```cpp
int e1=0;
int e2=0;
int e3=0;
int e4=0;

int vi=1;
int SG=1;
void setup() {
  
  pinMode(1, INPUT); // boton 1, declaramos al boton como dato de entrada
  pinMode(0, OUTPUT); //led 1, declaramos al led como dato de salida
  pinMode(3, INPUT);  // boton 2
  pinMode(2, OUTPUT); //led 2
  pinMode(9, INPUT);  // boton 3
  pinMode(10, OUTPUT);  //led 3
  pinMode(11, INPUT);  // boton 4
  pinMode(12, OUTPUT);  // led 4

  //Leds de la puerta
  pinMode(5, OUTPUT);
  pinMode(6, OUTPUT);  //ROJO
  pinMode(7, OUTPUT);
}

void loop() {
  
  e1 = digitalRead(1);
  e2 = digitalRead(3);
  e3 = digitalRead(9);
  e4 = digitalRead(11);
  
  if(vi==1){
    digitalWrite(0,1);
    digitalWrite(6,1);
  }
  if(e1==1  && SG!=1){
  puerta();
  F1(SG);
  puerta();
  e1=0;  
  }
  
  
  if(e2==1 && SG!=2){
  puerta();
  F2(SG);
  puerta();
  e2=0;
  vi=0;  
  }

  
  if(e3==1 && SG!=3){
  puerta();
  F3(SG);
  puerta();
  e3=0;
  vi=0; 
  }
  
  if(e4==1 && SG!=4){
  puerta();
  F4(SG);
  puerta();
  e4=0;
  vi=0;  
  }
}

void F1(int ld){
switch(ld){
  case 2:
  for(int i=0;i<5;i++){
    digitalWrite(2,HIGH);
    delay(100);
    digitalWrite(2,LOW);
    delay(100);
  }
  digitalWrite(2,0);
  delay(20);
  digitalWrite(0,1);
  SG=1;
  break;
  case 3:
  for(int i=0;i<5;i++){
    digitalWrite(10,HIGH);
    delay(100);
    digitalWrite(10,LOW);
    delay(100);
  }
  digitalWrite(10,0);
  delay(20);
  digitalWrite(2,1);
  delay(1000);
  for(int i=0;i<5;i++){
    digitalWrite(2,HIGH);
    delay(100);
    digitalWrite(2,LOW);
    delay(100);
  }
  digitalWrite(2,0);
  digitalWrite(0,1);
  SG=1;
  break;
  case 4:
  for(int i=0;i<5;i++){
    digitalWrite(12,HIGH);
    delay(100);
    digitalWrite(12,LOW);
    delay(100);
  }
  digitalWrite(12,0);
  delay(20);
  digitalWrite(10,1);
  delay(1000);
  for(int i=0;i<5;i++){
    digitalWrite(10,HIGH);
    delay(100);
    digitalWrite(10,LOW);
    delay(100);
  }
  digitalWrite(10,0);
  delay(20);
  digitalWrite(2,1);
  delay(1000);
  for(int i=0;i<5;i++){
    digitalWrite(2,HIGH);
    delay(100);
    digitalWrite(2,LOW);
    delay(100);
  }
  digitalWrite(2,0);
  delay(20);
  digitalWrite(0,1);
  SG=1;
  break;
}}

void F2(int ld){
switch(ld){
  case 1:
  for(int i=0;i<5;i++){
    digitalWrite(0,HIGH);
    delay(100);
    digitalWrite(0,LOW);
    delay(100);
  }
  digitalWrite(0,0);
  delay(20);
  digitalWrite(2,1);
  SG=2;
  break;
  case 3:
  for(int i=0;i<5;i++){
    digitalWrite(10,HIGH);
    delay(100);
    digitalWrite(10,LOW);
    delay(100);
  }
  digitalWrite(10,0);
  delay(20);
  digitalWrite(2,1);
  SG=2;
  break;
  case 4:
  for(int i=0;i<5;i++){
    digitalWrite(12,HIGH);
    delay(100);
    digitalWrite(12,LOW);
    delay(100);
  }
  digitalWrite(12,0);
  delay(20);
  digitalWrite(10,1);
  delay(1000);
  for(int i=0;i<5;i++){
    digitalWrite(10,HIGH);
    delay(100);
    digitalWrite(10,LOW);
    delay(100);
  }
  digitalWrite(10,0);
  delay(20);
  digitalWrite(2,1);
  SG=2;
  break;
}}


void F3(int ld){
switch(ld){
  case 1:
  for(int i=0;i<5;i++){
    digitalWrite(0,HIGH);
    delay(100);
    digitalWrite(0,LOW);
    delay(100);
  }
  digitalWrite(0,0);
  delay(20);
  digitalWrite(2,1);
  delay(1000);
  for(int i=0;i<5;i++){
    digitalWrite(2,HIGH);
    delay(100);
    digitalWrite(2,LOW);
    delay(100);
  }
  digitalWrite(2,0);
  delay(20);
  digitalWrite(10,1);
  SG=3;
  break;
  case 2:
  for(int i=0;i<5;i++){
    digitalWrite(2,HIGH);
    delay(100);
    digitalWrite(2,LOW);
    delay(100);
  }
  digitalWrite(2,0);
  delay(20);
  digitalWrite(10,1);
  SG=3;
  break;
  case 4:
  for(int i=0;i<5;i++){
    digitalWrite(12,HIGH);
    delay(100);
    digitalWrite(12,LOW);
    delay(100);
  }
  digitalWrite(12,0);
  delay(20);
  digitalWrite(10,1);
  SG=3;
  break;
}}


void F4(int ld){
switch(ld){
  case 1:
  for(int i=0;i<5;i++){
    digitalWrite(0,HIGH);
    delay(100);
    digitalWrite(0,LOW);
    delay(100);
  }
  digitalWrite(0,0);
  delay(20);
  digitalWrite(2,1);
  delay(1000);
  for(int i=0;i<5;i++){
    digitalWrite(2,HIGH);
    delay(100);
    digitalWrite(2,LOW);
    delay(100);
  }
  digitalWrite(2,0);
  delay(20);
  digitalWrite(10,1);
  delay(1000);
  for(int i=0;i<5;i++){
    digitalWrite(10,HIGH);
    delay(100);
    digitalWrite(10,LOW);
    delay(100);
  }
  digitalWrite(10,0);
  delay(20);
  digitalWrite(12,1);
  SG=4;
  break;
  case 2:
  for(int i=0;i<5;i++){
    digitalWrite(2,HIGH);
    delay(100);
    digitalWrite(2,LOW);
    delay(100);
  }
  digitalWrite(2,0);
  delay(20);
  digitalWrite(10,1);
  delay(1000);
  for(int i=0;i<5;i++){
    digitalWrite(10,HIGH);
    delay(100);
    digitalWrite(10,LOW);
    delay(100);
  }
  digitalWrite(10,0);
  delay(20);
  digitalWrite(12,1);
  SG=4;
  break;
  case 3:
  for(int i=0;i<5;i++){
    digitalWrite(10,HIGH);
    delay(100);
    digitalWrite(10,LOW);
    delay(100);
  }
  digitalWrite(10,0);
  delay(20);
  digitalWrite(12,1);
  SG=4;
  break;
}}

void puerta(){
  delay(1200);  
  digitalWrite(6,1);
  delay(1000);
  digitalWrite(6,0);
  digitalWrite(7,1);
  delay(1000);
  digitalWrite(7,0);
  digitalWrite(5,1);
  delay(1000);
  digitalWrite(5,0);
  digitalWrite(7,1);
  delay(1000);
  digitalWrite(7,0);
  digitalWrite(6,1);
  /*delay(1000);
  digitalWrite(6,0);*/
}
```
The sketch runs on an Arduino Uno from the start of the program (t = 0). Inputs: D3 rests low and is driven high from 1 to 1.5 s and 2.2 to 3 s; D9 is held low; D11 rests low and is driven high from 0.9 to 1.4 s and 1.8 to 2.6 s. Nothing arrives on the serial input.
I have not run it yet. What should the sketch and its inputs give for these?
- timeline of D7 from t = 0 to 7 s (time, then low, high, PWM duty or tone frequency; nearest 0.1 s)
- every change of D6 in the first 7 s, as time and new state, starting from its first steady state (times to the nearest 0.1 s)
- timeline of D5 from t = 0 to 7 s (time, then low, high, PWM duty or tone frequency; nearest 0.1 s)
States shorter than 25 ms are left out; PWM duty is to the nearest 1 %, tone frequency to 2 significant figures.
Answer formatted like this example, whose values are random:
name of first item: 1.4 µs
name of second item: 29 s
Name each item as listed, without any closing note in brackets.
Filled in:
timeline of D7 from t = 0 to 7 s: 0 s low; 3.1 s high; 4.1 s low; 5.1 s high; 6.1 s low
every change of D6 in the first 7 s, as time and new state, starting from its first steady state: 0 s high; 3.1 s low; 6.1 s high
timeline of D5 from t = 0 to 7 s: 0 s low; 4.1 s high; 5.1 s low
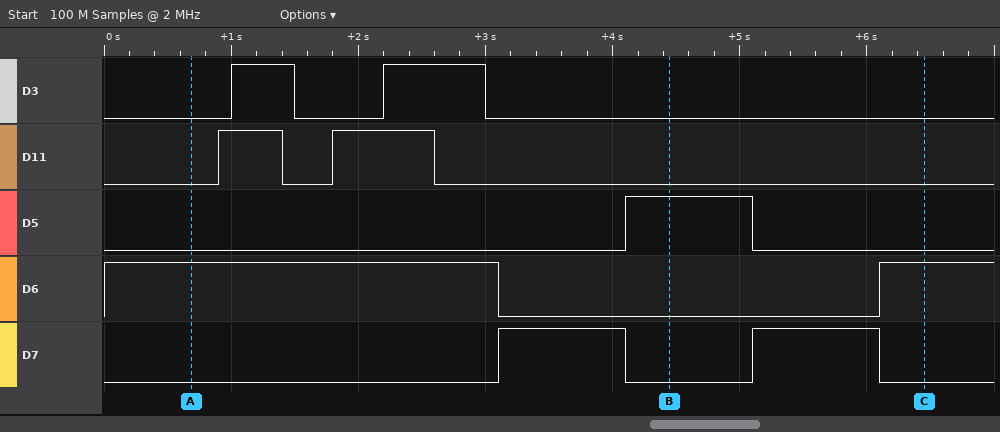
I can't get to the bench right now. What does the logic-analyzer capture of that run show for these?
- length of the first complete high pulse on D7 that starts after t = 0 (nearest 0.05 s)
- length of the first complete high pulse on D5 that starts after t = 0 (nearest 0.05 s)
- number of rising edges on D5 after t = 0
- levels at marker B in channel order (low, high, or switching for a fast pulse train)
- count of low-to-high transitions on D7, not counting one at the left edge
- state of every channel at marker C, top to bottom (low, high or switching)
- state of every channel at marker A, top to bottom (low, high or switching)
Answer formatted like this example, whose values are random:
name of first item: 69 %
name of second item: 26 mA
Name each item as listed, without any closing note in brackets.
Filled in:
length of the first complete high pulse on D7 that starts after t = 0: 1.00 s
length of the first complete high pulse on D5 that starts after t = 0: 1.00 s
number of rising edges on D5 after t = 0: 1
levels at marker B in channel order: D3 low, D11 low, D5 high, D6 low, D7 low
count of low-to-high transitions on D7, not counting one at the left edge: 2
state of every channel at marker C, top to bottom: D3 low, D11 low, D5 low, D6 high, D7 low
state of every channel at marker A, top to bottom: D3 low, D11 low, D5 low, D6 high, D7 low
